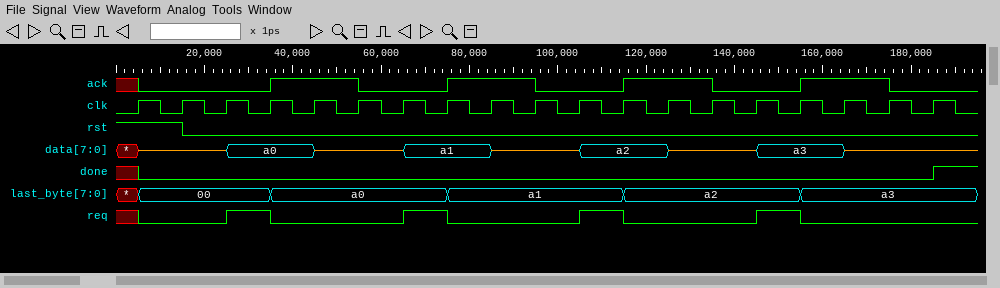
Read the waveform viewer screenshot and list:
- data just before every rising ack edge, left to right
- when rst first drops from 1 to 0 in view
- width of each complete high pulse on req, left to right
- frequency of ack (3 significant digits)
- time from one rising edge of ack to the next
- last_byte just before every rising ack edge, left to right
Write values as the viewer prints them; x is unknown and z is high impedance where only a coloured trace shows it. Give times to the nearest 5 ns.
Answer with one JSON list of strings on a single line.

["a0, a1, a2, a3", "15 ns", "10 ns, 10 ns, 10 ns, 10 ns", "25.0 MHz", "40 ns", "00, a0, a1, a2"]
